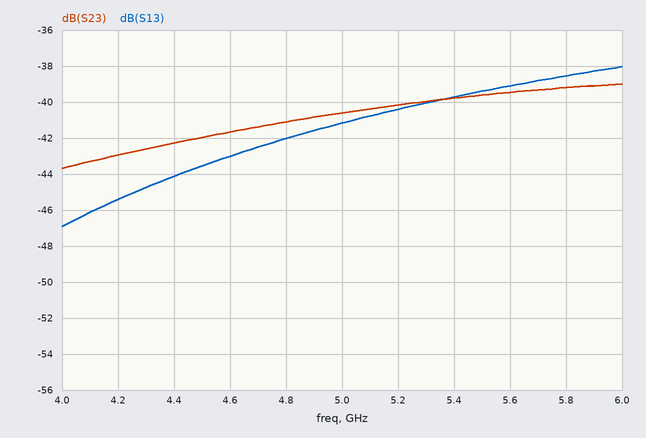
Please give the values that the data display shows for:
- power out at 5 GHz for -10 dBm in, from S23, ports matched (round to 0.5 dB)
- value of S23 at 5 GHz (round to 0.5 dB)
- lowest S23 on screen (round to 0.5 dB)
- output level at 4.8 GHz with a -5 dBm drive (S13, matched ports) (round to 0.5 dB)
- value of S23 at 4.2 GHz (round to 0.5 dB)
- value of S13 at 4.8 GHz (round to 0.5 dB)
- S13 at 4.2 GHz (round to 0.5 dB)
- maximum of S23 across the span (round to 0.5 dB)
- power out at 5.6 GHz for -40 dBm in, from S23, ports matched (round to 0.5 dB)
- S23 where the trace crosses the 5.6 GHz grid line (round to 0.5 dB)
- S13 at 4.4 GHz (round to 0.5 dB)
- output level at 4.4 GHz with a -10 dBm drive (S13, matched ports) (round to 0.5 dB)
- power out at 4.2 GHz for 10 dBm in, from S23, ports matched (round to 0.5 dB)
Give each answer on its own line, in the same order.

-50.5 dBm
-40.5 dB
-43.5 dB
-47.0 dBm
-43.0 dB
-42.0 dB
-45.5 dB
-39.0 dB
-79.5 dBm
-39.5 dB
-44.0 dB
-54.0 dBm
-33.0 dBm
